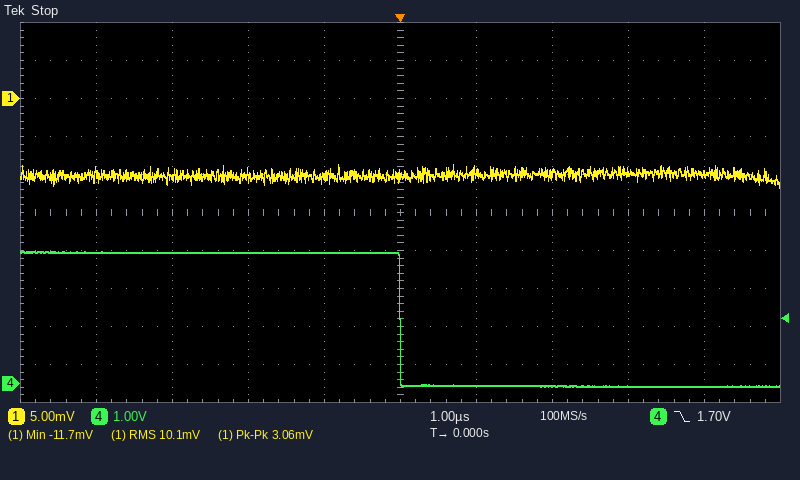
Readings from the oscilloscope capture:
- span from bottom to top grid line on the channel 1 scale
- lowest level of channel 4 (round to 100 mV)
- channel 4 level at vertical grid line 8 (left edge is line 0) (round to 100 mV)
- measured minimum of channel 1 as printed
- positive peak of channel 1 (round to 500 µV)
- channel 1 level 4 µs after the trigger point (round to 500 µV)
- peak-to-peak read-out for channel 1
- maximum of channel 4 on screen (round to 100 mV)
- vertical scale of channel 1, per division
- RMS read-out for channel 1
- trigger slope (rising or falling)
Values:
50 mV
-100 mV
-100 mV
-11.7 mV
-8.5 mV
-10.0 mV
3.06 mV
3.5 V
5 mV
10.1 mV
falling
